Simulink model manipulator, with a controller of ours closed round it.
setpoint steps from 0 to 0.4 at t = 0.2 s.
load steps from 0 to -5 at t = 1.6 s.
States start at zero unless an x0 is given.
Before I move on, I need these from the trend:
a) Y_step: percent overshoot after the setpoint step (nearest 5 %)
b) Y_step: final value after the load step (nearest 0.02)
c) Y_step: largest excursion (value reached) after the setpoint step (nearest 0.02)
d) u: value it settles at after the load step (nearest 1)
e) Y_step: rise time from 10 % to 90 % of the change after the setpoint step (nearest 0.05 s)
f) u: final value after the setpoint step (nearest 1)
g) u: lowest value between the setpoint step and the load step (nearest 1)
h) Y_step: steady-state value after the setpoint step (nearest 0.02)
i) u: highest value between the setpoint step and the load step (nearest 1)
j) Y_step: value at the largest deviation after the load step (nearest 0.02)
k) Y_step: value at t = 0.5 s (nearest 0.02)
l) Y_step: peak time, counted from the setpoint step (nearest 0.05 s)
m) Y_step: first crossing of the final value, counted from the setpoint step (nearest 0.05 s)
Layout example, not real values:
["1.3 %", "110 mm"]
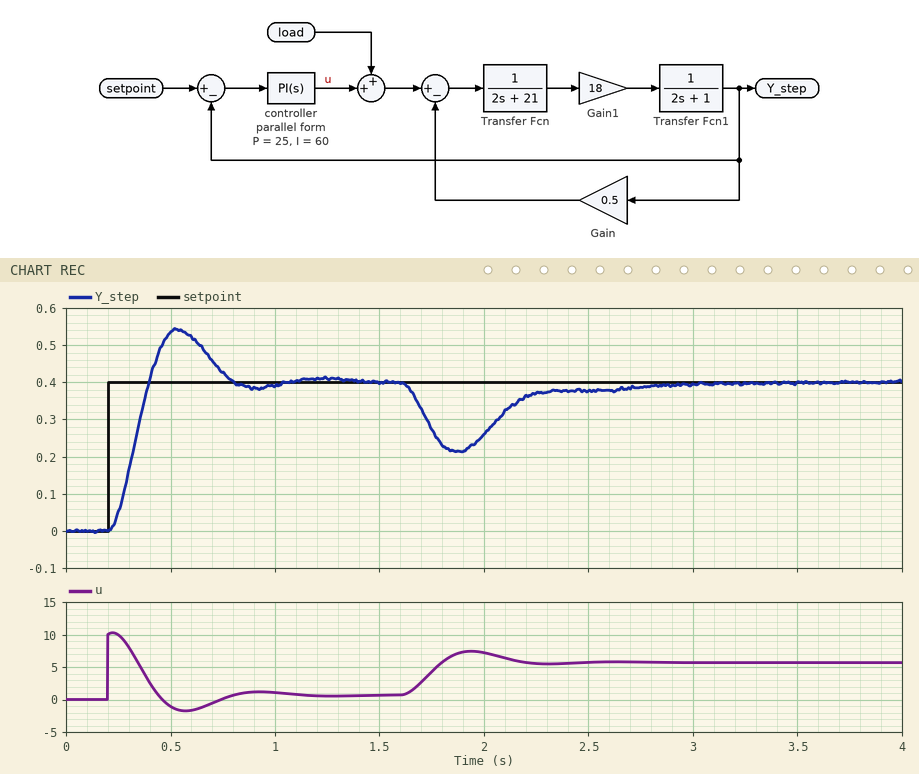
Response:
["35 %", "0.40", "0.54", "6", "0.15 s", "1", "-2", "0.40", "10", "0.22", "0.54", "0.35 s", "0.20 s"]
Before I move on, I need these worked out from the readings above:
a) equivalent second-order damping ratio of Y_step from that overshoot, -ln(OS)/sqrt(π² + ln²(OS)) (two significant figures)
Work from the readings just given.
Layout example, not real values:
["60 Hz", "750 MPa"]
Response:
["0.32"]
